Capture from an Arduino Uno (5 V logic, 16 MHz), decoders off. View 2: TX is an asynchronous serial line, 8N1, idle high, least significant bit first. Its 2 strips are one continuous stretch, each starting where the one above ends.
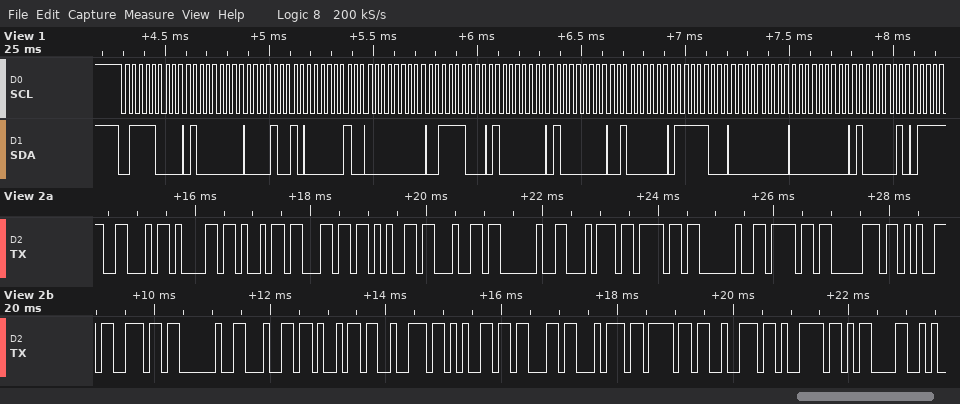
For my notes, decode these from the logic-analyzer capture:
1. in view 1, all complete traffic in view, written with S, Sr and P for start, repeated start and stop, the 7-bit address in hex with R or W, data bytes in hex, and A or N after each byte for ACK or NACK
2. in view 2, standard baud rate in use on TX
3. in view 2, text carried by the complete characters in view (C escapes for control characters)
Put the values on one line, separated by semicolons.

S 3CW A 40 A 09 A 02 A 00 A 3C A 40 A 40 A 20 A 7C A 00 A 00 A 41 A; 9600 baud; "Failed to open directory\r"
